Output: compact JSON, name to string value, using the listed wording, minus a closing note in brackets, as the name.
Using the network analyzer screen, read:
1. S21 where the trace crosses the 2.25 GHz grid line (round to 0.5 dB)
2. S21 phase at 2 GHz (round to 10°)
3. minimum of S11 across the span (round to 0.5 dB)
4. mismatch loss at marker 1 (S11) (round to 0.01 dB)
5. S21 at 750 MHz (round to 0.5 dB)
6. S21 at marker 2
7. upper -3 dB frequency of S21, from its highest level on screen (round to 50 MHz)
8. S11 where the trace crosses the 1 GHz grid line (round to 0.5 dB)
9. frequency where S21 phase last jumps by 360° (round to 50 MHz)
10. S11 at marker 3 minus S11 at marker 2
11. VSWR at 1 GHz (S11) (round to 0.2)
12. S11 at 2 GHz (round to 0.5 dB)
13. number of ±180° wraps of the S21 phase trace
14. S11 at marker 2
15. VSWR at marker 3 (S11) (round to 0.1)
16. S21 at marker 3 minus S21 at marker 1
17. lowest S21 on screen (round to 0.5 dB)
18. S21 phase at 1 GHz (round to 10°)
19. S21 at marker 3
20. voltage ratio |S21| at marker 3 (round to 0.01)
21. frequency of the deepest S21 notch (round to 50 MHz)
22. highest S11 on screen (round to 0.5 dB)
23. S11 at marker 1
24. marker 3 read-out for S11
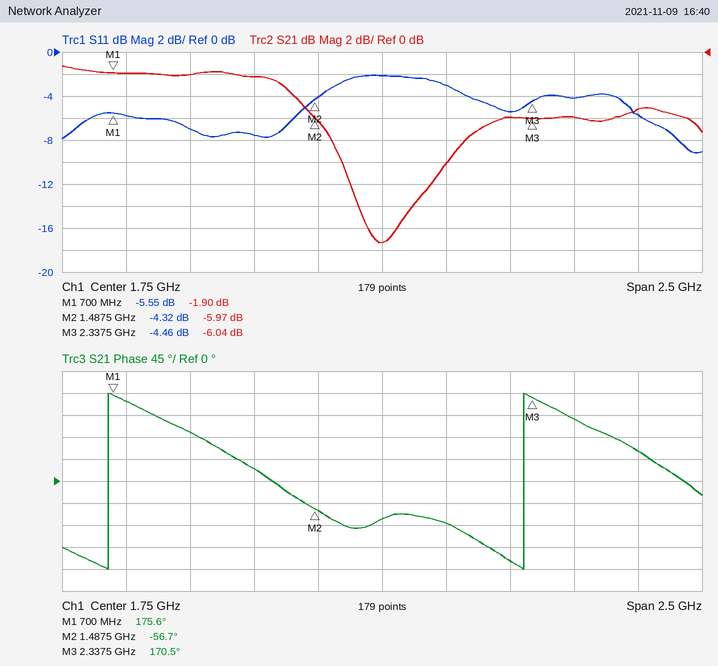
{"S21 where the trace crosses the 2.25 GHz grid line": "-6.0 dB", "S21 phase at 2 GHz": "-90°", "minimum of S11 across the span": "-9.0 dB", "mismatch loss at marker 1 (S11)": "1.42 dB", "S21 at 750 MHz": "-2.0 dB", "S21 at marker 2": "-5.97 dB", "upper -3 dB frequency of S21, from its highest level on screen": "1.40 GHz", "S11 where the trace crosses the 1 GHz grid line": "-7.0 dB", "frequency where S21 phase last jumps by 360°": "2.30 GHz", "S11 at marker 3 minus S11 at marker 2": "-0.14 dB", "VSWR at 1 GHz (S11)": "2.6", "S11 at 2 GHz": "-3.0 dB", "number of ±180° wraps of the S21 phase trace": "2", "S11 at marker 2": "-4.32 dB", "VSWR at marker 3 (S11)": "4.0", "S21 at marker 3 minus S21 at marker 1": "-4.14 dB", "lowest S21 on screen": "-17.5 dB", "S21 phase at 1 GHz": "100°", "S21 at marker 3": "-6.04 dB", "voltage ratio |S21| at marker 3": "0.50", "frequency of the deepest S21 notch": "1.75 GHz", "highest S11 on screen": "-2.0 dB", "S11 at marker 1": "-5.55 dB", "marker 3 read-out for S11": "-4.46 dB"}
